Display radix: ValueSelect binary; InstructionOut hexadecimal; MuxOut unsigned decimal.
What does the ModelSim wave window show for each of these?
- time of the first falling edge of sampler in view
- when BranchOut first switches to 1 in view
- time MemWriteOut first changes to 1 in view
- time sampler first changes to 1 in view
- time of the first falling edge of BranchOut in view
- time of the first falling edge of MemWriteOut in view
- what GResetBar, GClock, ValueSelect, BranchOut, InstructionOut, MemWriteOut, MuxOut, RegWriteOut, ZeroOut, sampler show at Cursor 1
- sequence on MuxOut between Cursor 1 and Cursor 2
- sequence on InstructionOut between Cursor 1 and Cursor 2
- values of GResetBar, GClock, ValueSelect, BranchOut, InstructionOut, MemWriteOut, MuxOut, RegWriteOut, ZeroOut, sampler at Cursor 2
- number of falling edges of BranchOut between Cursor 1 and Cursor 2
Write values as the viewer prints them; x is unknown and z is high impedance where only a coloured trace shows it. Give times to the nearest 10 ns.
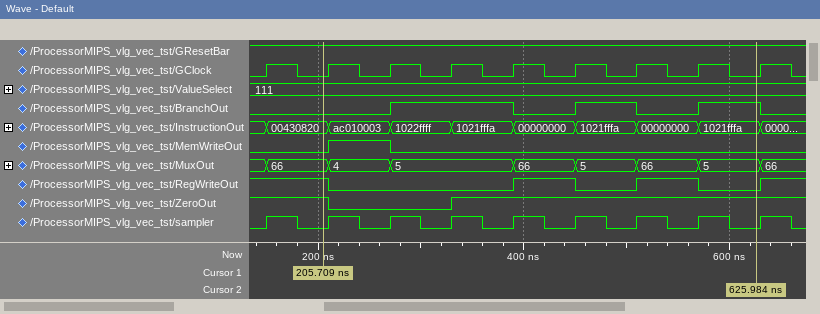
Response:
180 ns
270 ns
210 ns
150 ns
390 ns
270 ns
GResetBar=1, GClock=0, ValueSelect=111, BranchOut=0, InstructionOut=00430820, MemWriteOut=0, MuxOut=66, RegWriteOut=1, ZeroOut=1, sampler=0
66, 4, 5, 66, 5, 66, 5
00430820, ac010003, 1022ffff, 1021fffa, 00000000, 1021fffa, 00000000, 1021fffa
GResetBar=1, GClock=0, ValueSelect=111, BranchOut=1, InstructionOut=1021fffa, MemWriteOut=0, MuxOut=5, RegWriteOut=0, ZeroOut=1, sampler=0
2
